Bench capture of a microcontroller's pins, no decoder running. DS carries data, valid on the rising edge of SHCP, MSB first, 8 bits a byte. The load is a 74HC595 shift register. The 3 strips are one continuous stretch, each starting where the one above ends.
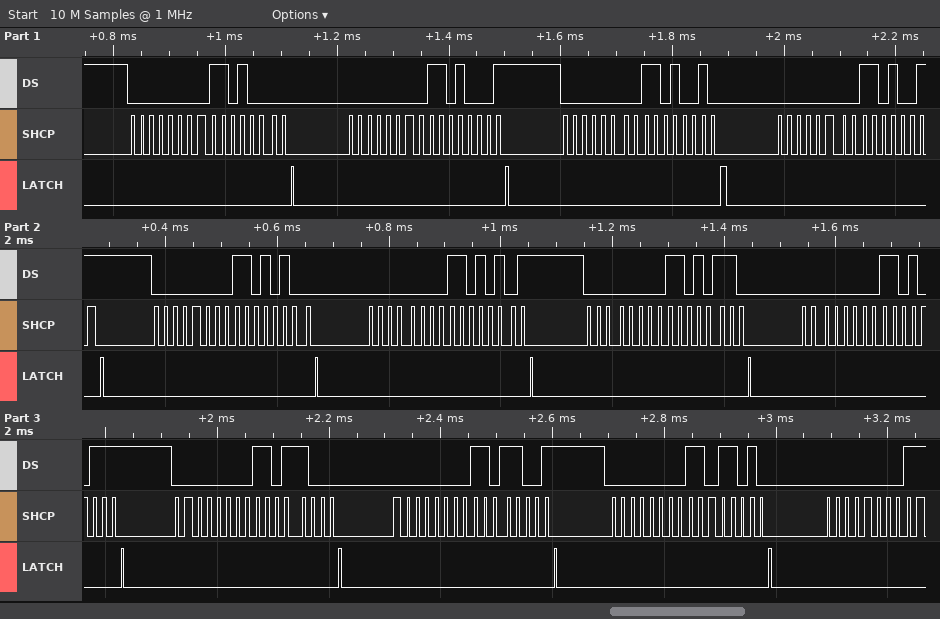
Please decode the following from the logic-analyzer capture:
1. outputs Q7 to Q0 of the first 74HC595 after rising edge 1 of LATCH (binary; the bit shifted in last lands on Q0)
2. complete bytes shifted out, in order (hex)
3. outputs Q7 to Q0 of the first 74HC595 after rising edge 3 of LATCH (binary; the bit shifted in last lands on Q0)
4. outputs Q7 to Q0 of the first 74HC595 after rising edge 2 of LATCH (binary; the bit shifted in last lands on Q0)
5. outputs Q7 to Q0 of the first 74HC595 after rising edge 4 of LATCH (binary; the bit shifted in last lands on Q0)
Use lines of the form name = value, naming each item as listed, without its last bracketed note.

outputs Q7 to Q0 of the first 74HC595 after rising edge 1 of LATCH = 11010000
complete bytes shifted out, in order = 00 D0 00 D1 00 D2 00 D3 00 D4 00 D5 00 D6 00 D7 00 D8 00 D9 00 DA 00
outputs Q7 to Q0 of the first 74HC595 after rising edge 3 of LATCH = 11010010
outputs Q7 to Q0 of the first 74HC595 after rising edge 2 of LATCH = 11010001
outputs Q7 to Q0 of the first 74HC595 after rising edge 4 of LATCH = 11010011
